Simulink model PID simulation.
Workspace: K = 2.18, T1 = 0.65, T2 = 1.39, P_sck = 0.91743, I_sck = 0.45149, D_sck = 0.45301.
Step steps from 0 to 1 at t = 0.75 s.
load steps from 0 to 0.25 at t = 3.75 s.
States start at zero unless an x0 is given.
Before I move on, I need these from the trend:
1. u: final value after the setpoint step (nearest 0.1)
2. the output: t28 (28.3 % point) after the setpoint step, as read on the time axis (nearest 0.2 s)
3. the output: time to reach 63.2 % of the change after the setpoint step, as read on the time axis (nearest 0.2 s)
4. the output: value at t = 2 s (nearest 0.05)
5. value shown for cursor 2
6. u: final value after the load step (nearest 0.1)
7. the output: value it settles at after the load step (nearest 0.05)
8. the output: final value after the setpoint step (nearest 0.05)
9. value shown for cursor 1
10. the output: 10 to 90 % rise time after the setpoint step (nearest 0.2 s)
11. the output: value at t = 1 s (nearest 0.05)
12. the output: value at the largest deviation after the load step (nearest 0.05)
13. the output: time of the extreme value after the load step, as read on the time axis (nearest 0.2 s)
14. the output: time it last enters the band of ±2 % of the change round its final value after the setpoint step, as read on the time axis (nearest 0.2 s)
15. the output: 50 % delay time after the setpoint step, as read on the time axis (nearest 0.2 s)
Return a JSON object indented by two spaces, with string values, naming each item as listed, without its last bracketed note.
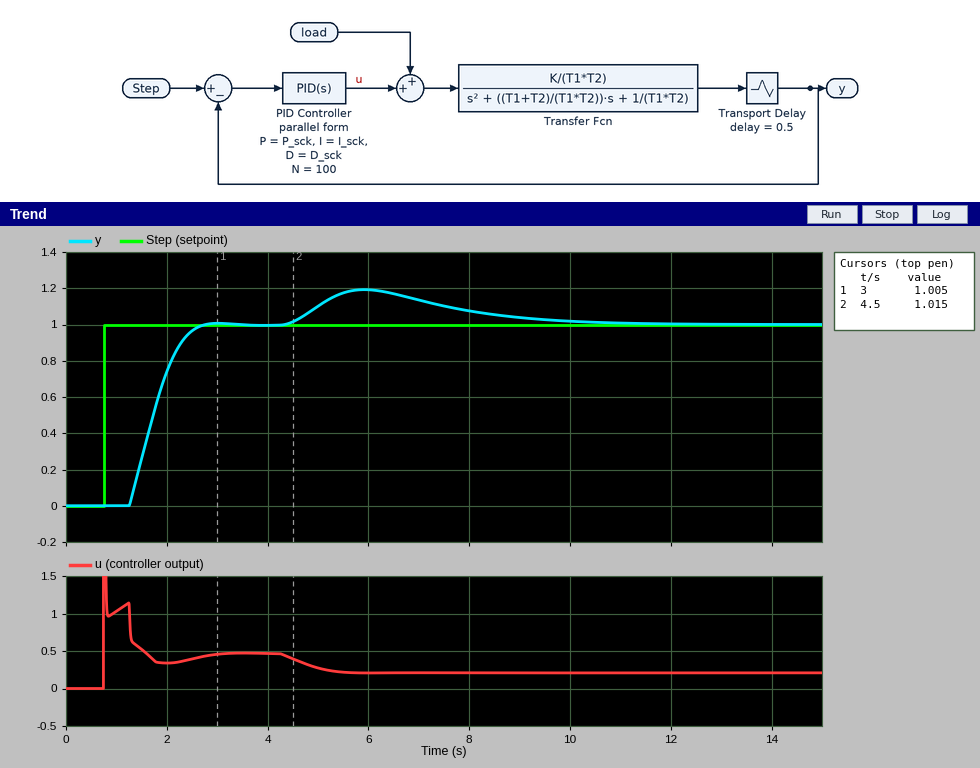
{
  "u: final value after the setpoint step": "0.5",
  "the output: t28 (28.3 % point) after the setpoint step, as read on the time axis": "1.6 s",
  "the output: time to reach 63.2 % of the change after the setpoint step, as read on the time axis": "1.8 s",
  "the output: value at t = 2 s": "0.75",
  "value shown for cursor 2": "1.015",
  "u: final value after the load step": "0.2",
  "the output: value it settles at after the load step": "1.00",
  "the output: final value after the setpoint step": "1.00",
  "value shown for cursor 1": "1.005",
  "the output: 10 to 90 % rise time after the setpoint step": "1.0 s",
  "the output: value at t = 1 s": "0.00",
  "the output: value at the largest deviation after the load step": "1.20",
  "the output: time of the extreme value after the load step, as read on the time axis": "6.0 s",
  "the output: time it last enters the band of ±2 % of the change round its final value after the setpoint step, as read on the time axis": "2.6 s",
  "the output: 50 % delay time after the setpoint step, as read on the time axis": "1.8 s"
}
